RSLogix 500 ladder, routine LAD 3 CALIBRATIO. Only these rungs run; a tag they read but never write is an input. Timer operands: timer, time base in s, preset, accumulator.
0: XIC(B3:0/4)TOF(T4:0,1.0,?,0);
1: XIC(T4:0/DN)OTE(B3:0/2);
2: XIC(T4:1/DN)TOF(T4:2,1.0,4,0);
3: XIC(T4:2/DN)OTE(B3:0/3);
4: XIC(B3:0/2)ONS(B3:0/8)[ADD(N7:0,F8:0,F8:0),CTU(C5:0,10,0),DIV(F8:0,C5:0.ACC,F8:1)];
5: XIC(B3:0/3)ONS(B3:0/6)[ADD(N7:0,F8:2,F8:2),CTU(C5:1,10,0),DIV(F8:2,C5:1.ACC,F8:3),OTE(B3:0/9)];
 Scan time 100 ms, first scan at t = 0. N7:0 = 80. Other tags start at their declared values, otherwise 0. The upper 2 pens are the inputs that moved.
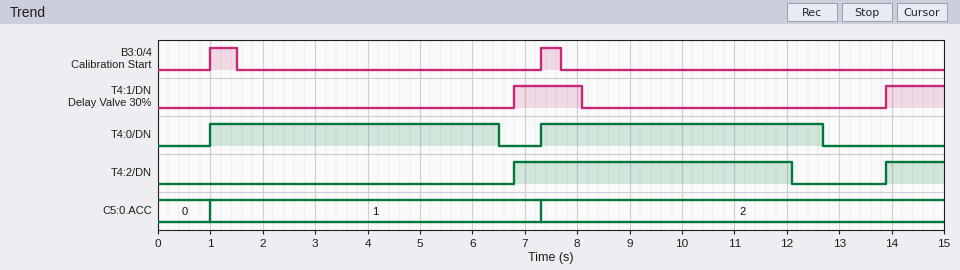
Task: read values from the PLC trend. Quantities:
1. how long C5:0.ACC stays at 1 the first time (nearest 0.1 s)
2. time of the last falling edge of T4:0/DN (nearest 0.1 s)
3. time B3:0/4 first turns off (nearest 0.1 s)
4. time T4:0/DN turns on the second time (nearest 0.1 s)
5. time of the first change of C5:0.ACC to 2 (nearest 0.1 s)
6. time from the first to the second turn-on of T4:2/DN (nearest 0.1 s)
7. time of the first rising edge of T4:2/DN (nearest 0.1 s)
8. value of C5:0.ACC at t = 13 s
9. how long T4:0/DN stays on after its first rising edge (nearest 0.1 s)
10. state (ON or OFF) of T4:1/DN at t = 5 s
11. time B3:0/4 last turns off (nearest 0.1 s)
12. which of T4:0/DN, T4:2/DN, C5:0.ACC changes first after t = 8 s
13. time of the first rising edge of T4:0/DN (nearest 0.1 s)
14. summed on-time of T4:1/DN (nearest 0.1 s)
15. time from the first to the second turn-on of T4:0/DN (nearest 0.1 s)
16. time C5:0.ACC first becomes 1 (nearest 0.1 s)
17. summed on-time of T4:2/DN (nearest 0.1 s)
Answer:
6.3 s
12.7 s
1.5 s
7.3 s
7.3 s
7.1 s
6.8 s
2
5.5 s
OFF
7.7 s
T4:2/DN
1.0 s
2.4 s
6.3 s
1.0 s
6.4 s
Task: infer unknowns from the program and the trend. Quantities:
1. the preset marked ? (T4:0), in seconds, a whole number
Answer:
5 s
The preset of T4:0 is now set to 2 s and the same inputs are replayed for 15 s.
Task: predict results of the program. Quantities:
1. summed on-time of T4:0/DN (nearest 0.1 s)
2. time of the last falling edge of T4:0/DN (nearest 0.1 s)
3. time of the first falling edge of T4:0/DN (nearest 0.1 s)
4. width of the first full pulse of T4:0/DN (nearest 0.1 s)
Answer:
4.9 s
9.7 s
3.5 s
2.5 s
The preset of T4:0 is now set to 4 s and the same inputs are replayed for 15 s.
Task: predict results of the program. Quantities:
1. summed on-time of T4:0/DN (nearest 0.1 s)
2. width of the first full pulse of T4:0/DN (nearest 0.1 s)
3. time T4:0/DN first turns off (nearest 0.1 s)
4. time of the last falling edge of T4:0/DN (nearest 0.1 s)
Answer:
8.9 s
4.5 s
5.5 s
11.7 s
